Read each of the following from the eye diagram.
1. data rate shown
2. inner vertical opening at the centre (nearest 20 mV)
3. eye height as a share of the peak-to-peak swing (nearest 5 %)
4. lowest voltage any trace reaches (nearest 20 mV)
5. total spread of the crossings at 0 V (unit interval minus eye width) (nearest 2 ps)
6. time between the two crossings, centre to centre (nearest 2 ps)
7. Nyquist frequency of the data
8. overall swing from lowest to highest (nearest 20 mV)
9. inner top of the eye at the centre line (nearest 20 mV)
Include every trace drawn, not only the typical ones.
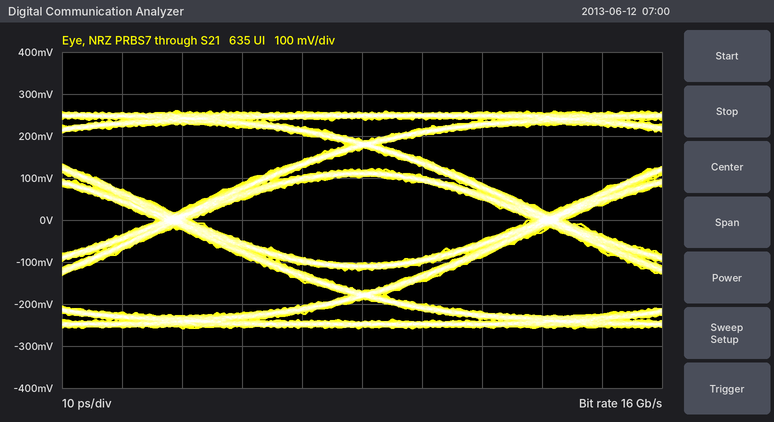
16 Gb/s
200 mV
40 %
-260 mV
6 ps
62 ps
8 GHz
520 mV
100 mV
